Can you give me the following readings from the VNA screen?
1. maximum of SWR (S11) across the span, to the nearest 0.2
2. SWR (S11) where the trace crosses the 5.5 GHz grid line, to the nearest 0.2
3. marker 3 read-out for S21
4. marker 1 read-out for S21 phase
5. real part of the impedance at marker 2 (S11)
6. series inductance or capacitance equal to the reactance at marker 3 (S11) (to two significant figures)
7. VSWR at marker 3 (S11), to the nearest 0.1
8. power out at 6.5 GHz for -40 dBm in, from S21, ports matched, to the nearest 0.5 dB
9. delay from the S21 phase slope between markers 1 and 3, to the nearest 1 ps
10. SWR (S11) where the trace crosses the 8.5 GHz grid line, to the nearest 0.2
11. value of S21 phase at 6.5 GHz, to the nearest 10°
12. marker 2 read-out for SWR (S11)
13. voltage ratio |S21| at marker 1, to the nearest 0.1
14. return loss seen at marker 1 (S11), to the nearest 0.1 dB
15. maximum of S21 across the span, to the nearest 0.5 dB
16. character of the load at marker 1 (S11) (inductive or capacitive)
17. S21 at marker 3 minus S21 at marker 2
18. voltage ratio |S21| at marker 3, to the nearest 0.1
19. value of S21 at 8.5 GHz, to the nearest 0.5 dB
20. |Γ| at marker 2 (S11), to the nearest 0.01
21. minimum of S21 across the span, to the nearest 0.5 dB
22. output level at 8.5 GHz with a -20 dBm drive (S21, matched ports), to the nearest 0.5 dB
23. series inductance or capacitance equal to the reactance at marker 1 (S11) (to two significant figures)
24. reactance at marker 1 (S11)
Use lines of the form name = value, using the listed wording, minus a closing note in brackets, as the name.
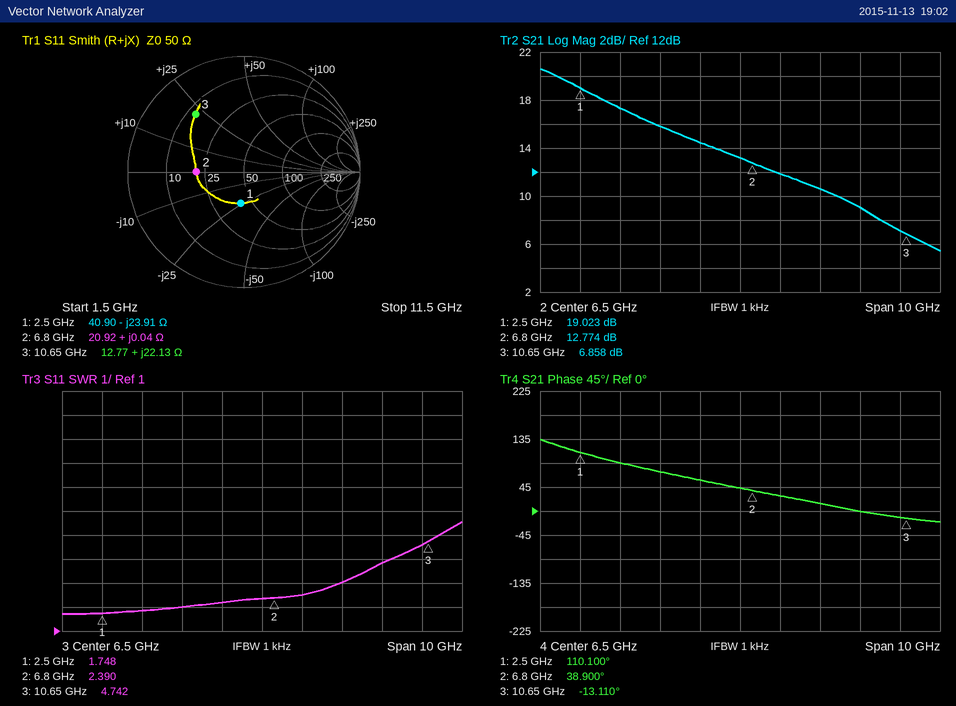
maximum of SWR (S11) across the span, to the nearest 0.2 = 5.6
SWR (S11) where the trace crosses the 5.5 GHz grid line, to the nearest 0.2 = 2.2
marker 3 read-out for S21 = 6.858 dB
marker 1 read-out for S21 phase = 110.100°
real part of the impedance at marker 2 = 20.92 Ω
series inductance or capacitance equal to the reactance at marker 3 (S11) = 330 pH
VSWR at marker 3 (S11), to the nearest 0.1 = 4.7
power out at 6.5 GHz for -40 dBm in, from S21, ports matched, to the nearest 0.5 dB = -27.0 dBm
delay from the S21 phase slope between markers 1 and 3, to the nearest 1 ps = 42 ps
SWR (S11) where the trace crosses the 8.5 GHz grid line, to the nearest 0.2 = 3.0
value of S21 phase at 6.5 GHz, to the nearest 10° = 40°
marker 2 read-out for SWR = 2.390
voltage ratio |S21| at marker 1, to the nearest 0.1 = 8.9
return loss seen at marker 1 (S11), to the nearest 0.1 dB = 11.3 dB
maximum of S21 across the span, to the nearest 0.5 dB = 20.5 dB
character of the load at marker 1 (S11) = capacitive
S21 at marker 3 minus S21 at marker 2 = -5.916 dB
voltage ratio |S21| at marker 3, to the nearest 0.1 = 2.2
value of S21 at 8.5 GHz, to the nearest 0.5 dB = 10.5 dB
|Γ| at marker 2 (S11), to the nearest 0.01 = 0.41
minimum of S21 across the span, to the nearest 0.5 dB = 5.5 dB
output level at 8.5 GHz with a -20 dBm drive (S21, matched ports), to the nearest 0.5 dB = -9.5 dBm
series inductance or capacitance equal to the reactance at marker 1 (S11) = 2.7 pF
reactance at marker 1 = -23.91 Ω
